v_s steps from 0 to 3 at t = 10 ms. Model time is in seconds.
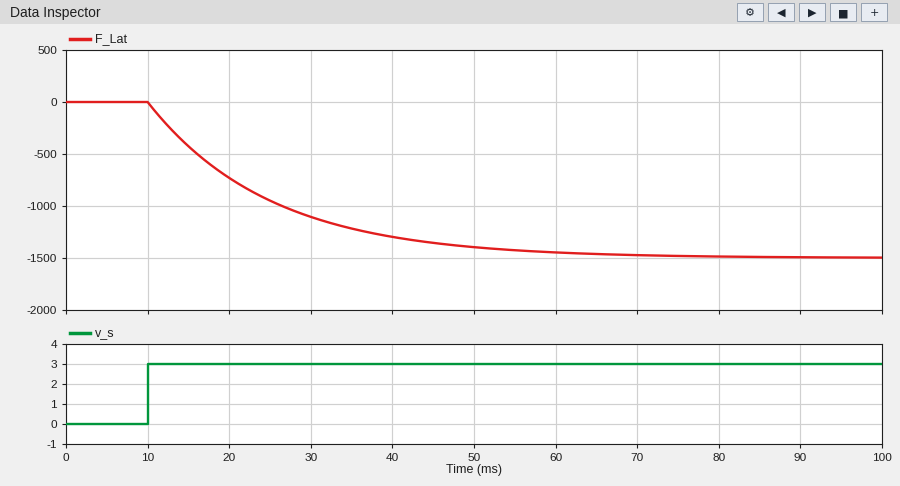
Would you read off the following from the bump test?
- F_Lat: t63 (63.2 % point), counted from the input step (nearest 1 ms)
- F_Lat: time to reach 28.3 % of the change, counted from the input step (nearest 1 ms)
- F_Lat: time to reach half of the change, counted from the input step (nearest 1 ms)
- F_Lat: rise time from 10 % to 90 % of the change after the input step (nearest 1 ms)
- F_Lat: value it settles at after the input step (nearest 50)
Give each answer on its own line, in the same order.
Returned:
15 ms
5 ms
10 ms
33 ms
-1500
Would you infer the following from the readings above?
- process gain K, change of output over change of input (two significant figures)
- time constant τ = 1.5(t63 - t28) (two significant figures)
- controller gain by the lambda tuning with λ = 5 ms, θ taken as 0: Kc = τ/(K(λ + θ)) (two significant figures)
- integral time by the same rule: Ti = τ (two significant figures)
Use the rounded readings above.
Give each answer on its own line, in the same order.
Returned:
-500
15 ms
-0.0060
15 ms
